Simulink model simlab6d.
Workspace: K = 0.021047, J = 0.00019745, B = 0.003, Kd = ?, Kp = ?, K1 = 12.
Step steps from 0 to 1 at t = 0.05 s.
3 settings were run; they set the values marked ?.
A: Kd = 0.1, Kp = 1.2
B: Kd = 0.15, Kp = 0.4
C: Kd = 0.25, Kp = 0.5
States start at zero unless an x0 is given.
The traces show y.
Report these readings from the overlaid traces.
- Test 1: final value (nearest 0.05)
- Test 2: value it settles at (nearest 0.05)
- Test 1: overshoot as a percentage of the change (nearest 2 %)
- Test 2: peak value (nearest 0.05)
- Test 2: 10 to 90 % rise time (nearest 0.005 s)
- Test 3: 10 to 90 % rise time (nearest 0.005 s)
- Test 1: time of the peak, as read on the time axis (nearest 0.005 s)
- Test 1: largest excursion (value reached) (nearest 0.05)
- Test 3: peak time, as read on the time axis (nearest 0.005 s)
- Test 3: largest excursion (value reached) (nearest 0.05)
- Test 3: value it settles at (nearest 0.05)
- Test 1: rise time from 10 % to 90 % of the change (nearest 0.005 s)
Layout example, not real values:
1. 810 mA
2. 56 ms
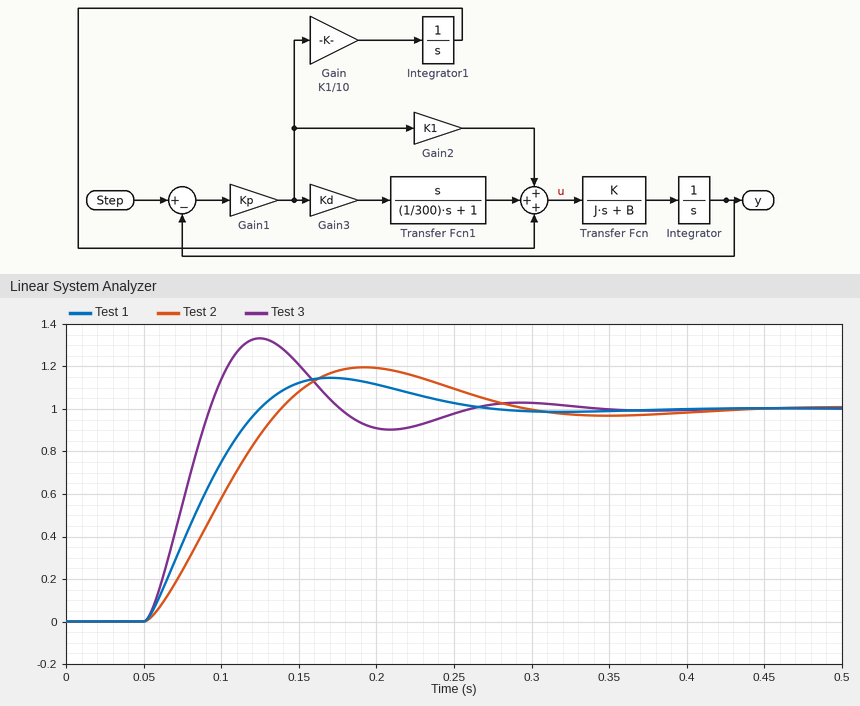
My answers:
1. 1.00
2. 1.00
3. 14 %
4. 1.20
5. 0.065 s
6. 0.030 s
7. 0.170 s
8. 1.15
9. 0.125 s
10. 1.35
11. 1.00
12. 0.055 s
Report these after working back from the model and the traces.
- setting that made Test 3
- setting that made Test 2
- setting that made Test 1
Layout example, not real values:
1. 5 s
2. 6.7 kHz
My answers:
1. A
2. B
3. C
